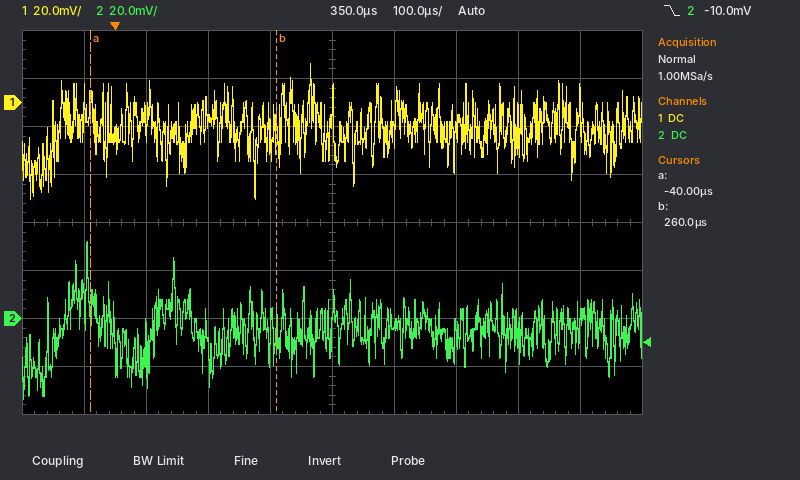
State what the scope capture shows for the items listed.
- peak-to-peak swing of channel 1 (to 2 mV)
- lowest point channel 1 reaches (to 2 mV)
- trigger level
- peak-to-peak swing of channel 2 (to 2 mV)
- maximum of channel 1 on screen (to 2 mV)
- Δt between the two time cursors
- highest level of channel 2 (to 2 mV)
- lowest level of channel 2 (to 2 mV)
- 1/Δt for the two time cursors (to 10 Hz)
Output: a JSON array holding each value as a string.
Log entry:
["56 mV", "-40 mV", "-10.0 mV", "66 mV", "16 mV", "300 µs", "32 mV", "-34 mV", "3.33 kHz"]
